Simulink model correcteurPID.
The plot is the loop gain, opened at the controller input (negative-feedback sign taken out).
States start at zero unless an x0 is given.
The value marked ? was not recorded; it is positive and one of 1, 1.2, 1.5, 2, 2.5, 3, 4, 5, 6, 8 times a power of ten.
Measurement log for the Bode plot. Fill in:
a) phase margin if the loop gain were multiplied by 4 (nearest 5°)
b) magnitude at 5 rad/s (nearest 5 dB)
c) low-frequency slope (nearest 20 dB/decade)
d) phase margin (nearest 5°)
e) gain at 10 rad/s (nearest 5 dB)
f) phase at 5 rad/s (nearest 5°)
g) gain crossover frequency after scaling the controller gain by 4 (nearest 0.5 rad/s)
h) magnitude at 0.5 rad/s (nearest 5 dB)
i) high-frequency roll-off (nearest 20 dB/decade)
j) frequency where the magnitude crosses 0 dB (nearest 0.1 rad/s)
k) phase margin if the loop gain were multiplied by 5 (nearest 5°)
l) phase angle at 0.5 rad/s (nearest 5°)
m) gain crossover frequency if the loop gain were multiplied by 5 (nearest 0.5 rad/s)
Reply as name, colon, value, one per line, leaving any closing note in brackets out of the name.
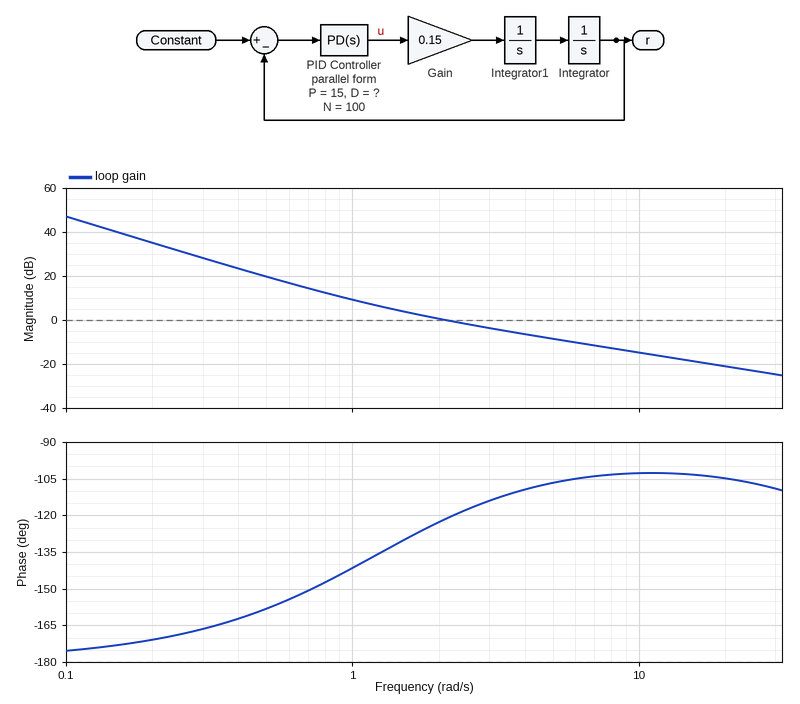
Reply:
phase margin if the loop gain were multiplied by 4: 75°
magnitude at 5 rad/s: -10 dB
low-frequency slope: -40 dB/decade
phase margin: 60°
gain at 10 rad/s: -15 dB
phase at 5 rad/s: -105°
gain crossover frequency after scaling the controller gain by 4: 7.5 rad/s
magnitude at 0.5 rad/s: 20 dB
high-frequency roll-off: -20 dB/decade
frequency where the magnitude crosses 0 dB: 2.1 rad/s
phase margin if the loop gain were multiplied by 5: 75°
phase angle at 0.5 rad/s: -160°
gain crossover frequency if the loop gain were multiplied by 5: 9.0 rad/s
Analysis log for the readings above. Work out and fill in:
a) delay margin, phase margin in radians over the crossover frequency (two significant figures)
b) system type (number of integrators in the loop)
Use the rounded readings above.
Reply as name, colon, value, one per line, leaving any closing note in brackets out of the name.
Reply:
delay margin, phase margin in radians over the crossover frequency: 0.50 s
system type: 2
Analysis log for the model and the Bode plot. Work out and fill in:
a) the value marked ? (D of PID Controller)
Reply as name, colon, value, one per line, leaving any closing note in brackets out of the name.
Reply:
the value marked ?: 12
